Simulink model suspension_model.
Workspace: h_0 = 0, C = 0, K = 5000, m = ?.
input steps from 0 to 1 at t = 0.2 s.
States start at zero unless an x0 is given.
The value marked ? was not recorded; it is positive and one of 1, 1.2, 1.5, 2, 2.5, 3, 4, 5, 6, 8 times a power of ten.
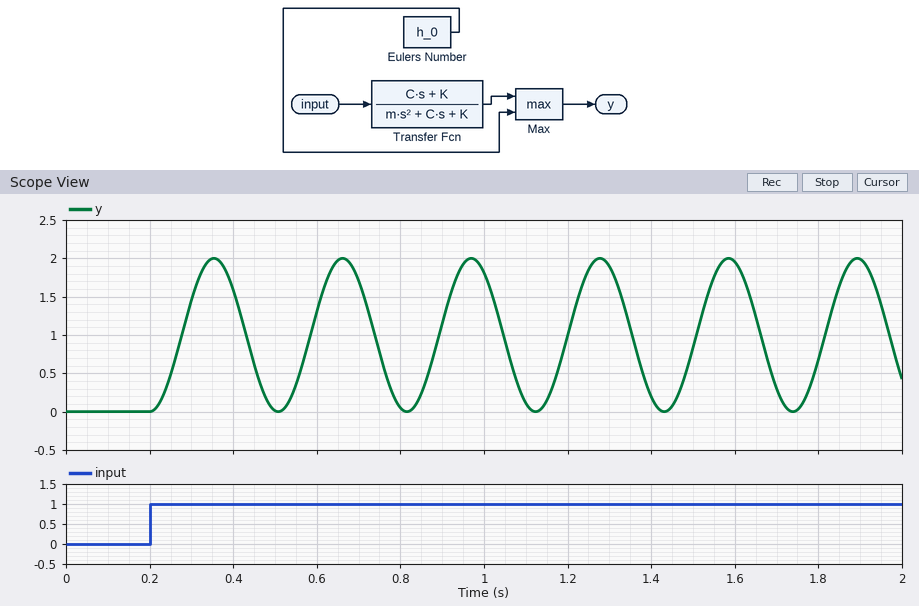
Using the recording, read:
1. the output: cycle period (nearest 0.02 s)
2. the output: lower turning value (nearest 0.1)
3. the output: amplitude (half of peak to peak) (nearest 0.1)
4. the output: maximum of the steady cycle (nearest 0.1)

0.30 s
0.0
1.0
2.0
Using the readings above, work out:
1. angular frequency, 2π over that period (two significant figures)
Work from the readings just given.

21 rad/s
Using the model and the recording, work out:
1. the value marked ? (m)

12
